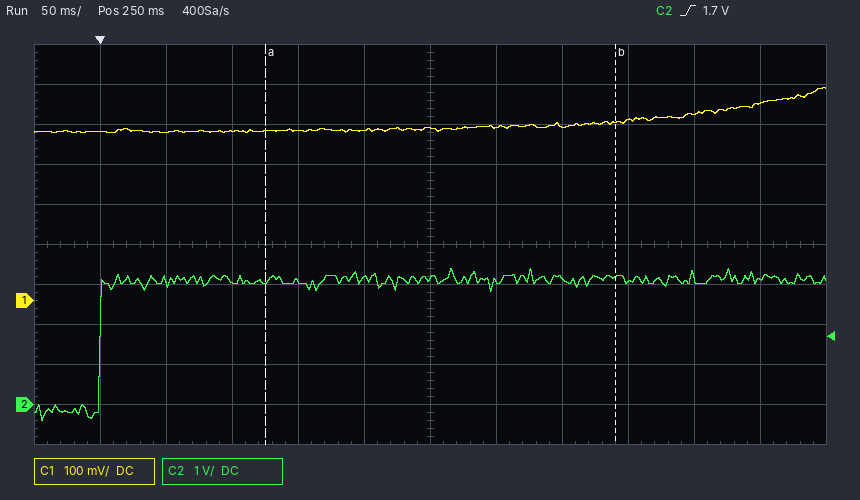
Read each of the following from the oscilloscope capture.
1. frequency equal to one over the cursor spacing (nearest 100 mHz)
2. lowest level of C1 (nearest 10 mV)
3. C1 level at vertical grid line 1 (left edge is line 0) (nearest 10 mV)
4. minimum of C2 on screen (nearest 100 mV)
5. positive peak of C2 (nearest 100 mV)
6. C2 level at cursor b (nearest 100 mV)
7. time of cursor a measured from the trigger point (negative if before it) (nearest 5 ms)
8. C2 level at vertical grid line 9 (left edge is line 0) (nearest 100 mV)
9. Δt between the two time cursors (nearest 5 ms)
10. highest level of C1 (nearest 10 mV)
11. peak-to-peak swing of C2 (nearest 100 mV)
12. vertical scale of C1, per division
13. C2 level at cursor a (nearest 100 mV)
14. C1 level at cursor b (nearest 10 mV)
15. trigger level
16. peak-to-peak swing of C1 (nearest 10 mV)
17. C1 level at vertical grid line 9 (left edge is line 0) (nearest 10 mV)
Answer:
3.8 Hz
420 mV
420 mV
-400 mV
3.4 V
3.2 V
+125 ms
3.1 V
265 ms
530 mV
3.8 V
100 mV
3.1 V
450 mV
1.7 V
110 mV
450 mV
